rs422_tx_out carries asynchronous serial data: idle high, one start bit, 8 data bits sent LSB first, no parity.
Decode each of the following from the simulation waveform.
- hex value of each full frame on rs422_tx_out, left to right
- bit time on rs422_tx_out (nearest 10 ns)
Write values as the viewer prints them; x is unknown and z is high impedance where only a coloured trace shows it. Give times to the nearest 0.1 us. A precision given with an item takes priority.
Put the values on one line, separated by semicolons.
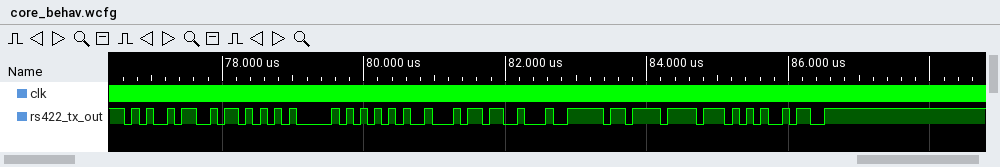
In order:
A5, 5A, 05, 55, A2, 13, BE, EF, 57, 9A; 100 ns
